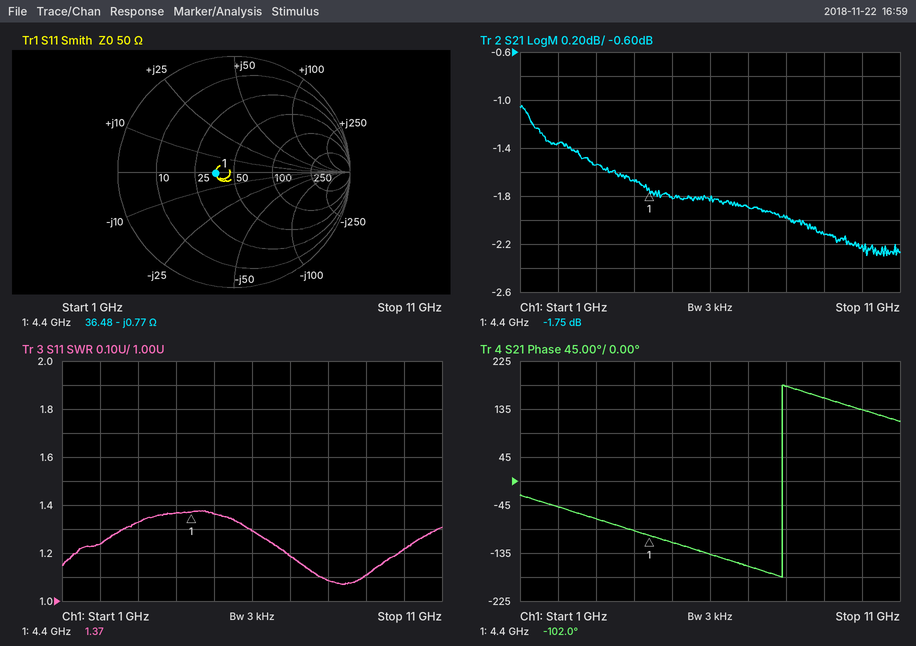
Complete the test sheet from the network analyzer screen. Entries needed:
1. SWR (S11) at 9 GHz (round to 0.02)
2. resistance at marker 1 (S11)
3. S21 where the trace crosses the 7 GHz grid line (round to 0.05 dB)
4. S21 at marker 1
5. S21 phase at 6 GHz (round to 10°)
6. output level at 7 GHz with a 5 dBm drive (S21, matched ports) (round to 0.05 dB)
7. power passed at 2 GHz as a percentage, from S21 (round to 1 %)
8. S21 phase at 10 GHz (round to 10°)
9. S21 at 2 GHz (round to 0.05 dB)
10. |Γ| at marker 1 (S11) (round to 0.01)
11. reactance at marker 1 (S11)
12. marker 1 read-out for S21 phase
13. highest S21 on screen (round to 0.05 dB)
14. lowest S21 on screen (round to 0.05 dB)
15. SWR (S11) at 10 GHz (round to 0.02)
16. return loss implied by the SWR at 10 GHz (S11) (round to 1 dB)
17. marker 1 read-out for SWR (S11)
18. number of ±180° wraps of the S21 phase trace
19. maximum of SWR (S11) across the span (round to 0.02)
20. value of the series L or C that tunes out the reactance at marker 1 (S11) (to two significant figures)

1.10
36.48 Ω
-1.90 dB
-1.75 dB
-140°
3.10 dBm
73 %
130°
-1.35 dB
0.16
-0.77 Ω
-102.0°
-1.05 dB
-2.30 dB
1.22
20 dB
1.37
1
1.38
28 pH
